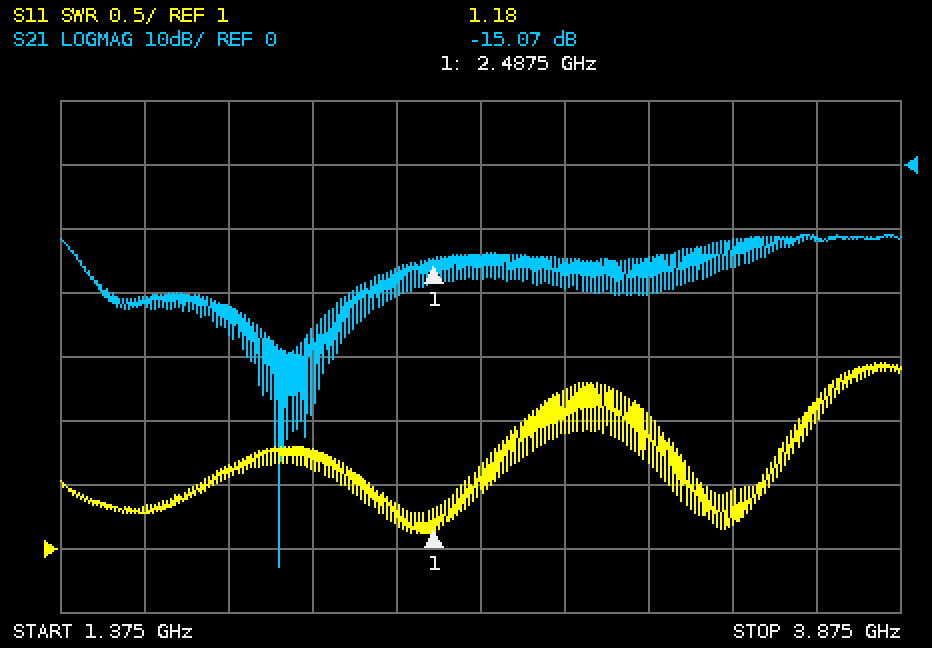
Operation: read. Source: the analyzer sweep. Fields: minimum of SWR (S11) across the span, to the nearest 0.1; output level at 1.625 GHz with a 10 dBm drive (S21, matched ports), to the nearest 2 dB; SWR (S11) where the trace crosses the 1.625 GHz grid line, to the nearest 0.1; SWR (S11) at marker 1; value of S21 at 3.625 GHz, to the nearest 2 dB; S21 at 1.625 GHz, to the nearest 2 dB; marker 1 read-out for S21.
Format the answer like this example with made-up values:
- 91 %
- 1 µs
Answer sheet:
- 1.1
- -12 dBm
- 1.3
- 1.18
- -12 dB
- -22 dB
- -15.07 dB
